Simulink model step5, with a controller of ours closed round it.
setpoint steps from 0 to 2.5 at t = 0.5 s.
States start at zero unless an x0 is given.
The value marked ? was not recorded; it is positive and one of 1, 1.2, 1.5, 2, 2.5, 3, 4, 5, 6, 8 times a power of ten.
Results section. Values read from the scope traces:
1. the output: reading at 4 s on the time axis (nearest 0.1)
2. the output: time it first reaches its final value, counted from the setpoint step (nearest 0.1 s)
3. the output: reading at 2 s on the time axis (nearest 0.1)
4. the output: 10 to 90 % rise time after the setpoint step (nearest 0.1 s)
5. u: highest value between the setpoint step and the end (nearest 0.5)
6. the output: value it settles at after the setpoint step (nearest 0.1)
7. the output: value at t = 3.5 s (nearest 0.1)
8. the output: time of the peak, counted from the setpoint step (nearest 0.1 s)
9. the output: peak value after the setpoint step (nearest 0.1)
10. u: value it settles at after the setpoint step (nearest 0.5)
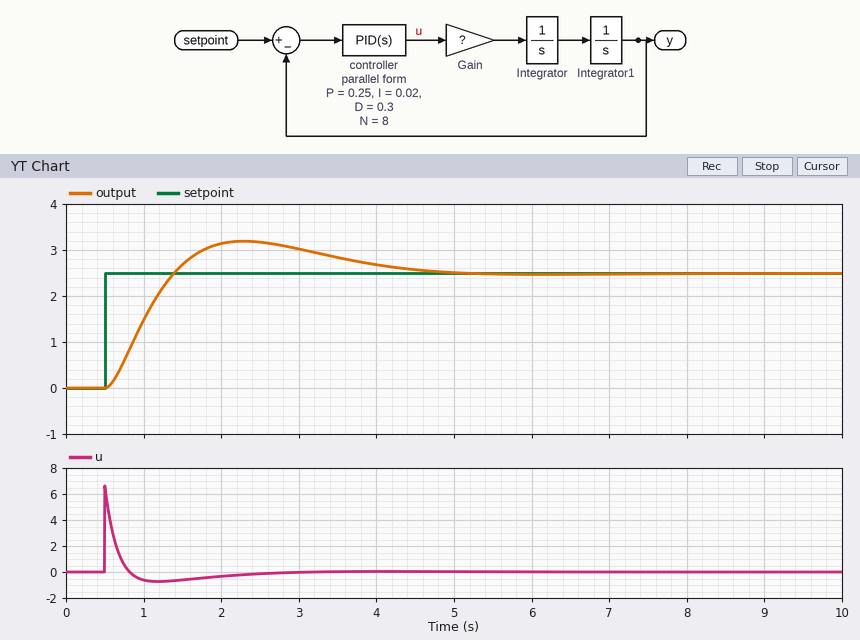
2.7
0.9 s
3.1
0.6 s
6.5
2.5
2.8
1.8 s
3.2
0.0
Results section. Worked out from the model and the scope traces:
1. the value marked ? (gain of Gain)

5
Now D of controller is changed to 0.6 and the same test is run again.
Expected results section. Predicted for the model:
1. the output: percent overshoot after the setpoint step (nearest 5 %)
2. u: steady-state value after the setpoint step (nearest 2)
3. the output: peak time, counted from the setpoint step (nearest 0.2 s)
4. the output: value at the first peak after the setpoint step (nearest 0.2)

15 %
0
1.0 s
2.8
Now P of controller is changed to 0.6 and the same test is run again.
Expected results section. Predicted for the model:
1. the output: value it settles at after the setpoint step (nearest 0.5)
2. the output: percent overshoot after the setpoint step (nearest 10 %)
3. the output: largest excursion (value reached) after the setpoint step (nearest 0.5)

2.5
40 %
3.5
